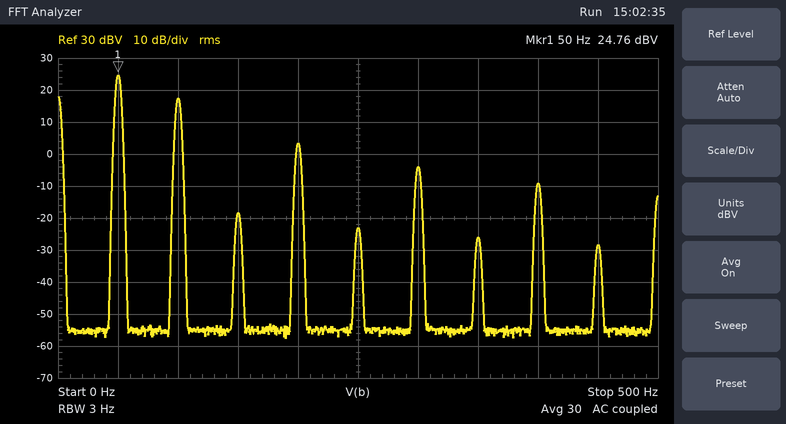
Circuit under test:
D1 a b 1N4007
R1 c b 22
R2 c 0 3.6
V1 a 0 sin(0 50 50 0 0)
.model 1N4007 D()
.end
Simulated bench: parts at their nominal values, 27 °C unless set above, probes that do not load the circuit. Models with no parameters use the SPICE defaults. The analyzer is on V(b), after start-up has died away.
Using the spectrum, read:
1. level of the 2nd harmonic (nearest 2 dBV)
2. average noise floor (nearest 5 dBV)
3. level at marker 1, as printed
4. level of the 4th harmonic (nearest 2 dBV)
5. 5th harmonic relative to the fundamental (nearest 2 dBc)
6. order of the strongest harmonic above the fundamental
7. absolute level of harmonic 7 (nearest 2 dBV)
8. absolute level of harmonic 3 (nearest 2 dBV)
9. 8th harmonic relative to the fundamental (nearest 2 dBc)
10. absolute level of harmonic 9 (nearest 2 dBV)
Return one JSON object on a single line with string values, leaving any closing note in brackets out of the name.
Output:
{"level of the 2nd harmonic": "18 dBV", "average noise floor": "-55 dBV", "level at marker 1, as printed": "24.76 dBV", "level of the 4th harmonic": "4 dBV", "5th harmonic relative to the fundamental": "-48 dBc", "order of the strongest harmonic above the fundamental": "2", "absolute level of harmonic 7": "-26 dBV", "absolute level of harmonic 3": "-18 dBV", "8th harmonic relative to the fundamental": "-34 dBc", "absolute level of harmonic 9": "-28 dBV"}
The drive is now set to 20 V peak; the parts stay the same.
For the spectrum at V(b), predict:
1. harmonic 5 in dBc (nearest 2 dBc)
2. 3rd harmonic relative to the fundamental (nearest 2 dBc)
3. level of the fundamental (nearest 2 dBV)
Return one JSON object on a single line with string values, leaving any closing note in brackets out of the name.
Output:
{"harmonic 5 in dBc": "-40 dBc", "3rd harmonic relative to the fundamental": "-36 dBc", "level of the fundamental": "16 dBV"}
